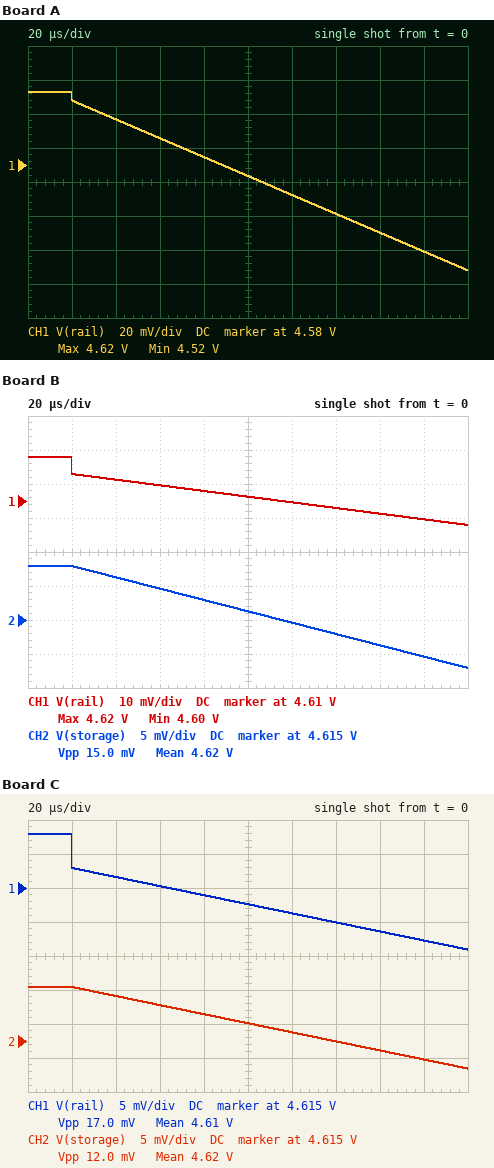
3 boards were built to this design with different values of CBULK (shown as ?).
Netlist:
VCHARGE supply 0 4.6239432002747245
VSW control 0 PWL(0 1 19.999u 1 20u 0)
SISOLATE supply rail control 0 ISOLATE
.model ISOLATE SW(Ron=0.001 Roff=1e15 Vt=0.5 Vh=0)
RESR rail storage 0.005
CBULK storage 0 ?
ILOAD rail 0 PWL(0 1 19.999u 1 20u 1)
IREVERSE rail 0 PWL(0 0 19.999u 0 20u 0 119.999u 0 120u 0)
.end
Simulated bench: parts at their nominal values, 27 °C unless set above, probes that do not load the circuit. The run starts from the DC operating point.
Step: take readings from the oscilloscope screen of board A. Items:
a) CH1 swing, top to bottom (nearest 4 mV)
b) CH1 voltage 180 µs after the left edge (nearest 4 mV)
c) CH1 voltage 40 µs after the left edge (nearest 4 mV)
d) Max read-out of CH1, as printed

104 mV
4.528 V
4.608 V
4.62 V
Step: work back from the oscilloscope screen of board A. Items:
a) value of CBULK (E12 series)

1.8 mF
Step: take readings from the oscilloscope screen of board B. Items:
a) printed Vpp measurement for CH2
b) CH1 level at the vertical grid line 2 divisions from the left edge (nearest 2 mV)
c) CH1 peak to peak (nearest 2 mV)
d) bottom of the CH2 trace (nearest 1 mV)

15.0 mV
4.616 V
20 mV
4.608 V
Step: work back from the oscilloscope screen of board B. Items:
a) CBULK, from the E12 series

12 mF
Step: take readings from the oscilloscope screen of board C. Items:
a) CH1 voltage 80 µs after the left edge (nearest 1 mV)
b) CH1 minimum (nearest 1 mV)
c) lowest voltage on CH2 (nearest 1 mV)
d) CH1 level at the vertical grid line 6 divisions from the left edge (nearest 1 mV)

4.614 V
4.606 V
4.611 V
4.611 V
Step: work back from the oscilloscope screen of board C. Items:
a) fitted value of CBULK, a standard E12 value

15 mF
